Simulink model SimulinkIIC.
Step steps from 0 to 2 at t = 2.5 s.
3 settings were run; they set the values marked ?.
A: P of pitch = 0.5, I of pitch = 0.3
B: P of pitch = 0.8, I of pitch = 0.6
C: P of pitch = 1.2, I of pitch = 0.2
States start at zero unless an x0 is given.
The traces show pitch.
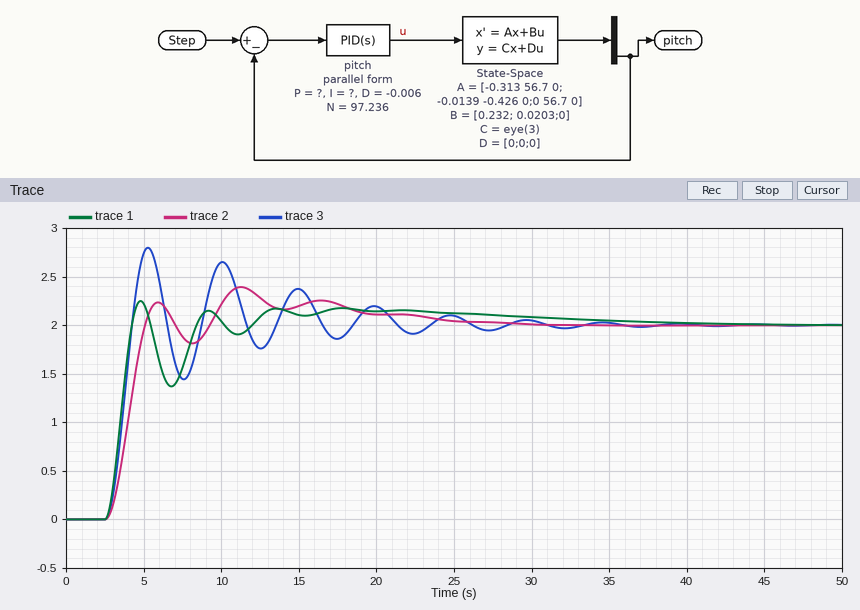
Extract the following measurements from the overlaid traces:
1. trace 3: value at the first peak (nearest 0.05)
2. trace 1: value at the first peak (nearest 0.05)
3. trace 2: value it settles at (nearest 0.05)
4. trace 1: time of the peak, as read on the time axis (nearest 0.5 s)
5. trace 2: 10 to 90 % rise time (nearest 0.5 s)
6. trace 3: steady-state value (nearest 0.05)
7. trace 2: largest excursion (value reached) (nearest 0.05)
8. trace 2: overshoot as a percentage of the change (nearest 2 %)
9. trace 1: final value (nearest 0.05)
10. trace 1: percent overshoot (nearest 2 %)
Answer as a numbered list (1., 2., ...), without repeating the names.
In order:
1. 2.80
2. 2.25
3. 2.00
4. 5.0 s
5. 1.5 s
6. 2.00
7. 2.40
8. 20 %
9. 2.00
10. 12 %
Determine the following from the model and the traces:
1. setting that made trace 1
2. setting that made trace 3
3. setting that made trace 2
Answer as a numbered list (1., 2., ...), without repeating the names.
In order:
1. C
2. B
3. A
